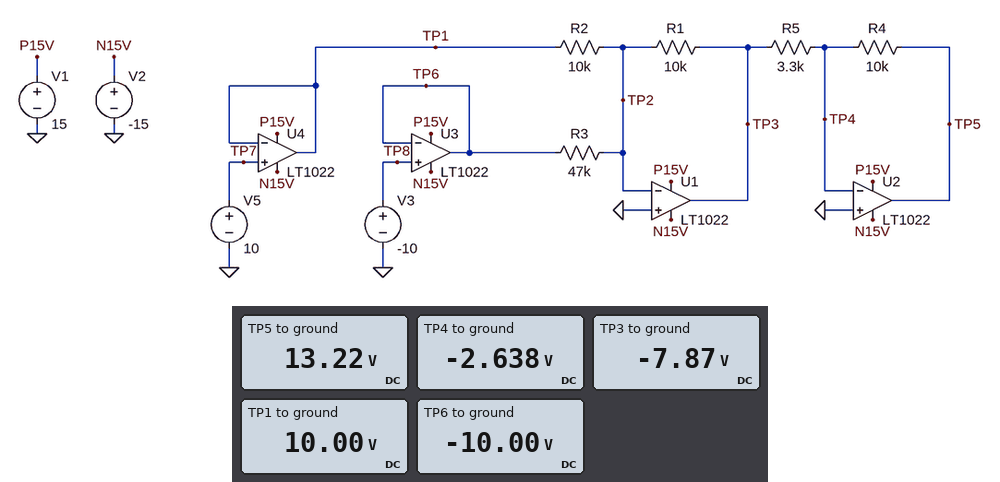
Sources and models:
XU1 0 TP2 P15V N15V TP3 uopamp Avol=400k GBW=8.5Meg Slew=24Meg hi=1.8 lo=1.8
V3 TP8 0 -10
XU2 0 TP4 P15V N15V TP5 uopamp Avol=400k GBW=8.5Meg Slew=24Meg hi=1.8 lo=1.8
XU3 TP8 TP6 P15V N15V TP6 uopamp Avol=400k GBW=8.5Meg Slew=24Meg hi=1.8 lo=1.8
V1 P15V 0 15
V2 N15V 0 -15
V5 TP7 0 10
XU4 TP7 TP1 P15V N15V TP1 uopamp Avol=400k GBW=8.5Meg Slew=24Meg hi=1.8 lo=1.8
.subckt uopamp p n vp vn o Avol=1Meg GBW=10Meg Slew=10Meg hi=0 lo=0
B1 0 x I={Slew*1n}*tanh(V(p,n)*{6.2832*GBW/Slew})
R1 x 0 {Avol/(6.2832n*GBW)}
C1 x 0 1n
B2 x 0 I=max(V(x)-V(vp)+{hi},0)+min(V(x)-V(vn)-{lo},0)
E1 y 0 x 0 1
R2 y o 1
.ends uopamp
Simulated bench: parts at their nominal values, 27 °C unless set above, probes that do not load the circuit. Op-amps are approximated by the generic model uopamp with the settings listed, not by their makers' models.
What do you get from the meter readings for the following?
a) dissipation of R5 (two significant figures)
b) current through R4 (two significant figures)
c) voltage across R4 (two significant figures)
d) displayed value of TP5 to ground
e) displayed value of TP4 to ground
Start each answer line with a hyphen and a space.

- 8.3 mW
- 1.6 mA
- 16 V
- 13.22 V
- -2.638 V
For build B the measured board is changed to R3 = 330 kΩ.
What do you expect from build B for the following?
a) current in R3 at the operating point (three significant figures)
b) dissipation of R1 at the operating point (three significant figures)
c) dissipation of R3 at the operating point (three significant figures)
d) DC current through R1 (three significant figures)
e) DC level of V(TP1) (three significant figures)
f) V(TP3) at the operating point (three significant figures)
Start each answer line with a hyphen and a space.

- 30.3 µA
- 9.40 mW
- 303 µW
- 970 µA
- 10.0 V
- -9.70 V
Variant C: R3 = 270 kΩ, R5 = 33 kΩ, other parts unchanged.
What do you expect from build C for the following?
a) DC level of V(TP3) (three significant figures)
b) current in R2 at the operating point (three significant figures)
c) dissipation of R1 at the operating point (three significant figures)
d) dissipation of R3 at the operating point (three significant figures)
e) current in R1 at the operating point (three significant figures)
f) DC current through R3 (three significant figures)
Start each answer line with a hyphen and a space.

- -9.63 V
- 1.00 mA
- 9.27 mW
- 370 µW
- 963 µA
- 37.0 µA
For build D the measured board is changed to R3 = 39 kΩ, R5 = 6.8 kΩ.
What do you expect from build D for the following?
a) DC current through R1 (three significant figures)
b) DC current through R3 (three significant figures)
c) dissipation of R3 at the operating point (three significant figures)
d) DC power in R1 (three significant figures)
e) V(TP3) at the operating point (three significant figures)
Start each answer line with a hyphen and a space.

- 744 µA
- 256 µA
- 2.56 mW
- 5.53 mW
- -7.44 V
